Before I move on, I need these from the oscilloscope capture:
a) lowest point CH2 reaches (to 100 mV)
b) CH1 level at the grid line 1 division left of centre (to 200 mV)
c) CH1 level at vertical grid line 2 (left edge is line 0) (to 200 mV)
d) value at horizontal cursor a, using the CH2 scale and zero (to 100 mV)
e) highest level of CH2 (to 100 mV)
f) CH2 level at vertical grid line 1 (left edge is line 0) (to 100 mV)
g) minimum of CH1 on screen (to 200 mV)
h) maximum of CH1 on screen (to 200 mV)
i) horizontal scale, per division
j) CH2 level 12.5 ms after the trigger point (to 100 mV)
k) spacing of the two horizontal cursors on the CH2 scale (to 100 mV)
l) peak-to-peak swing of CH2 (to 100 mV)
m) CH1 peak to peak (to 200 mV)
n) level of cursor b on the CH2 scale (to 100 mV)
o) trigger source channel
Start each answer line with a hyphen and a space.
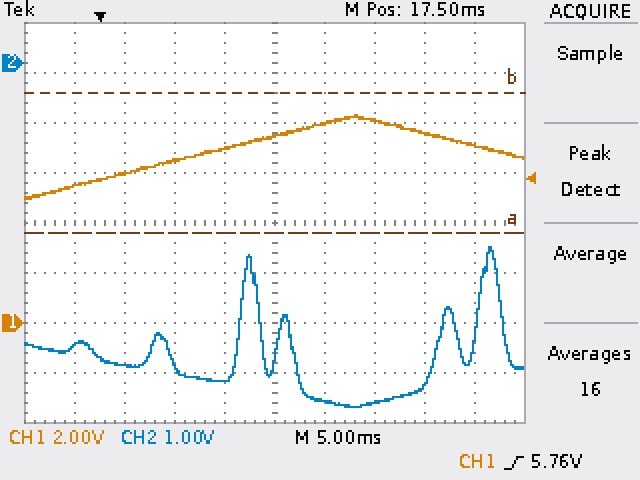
- -6.9 V
- 7.0 V
- 6.0 V
- -3.4 V
- -3.7 V
- -5.7 V
- 5.0 V
- 8.4 V
- 5 ms
- -6.4 V
- 2.8 V
- 3.2 V
- 3.4 V
- -600 mV
- CH1
